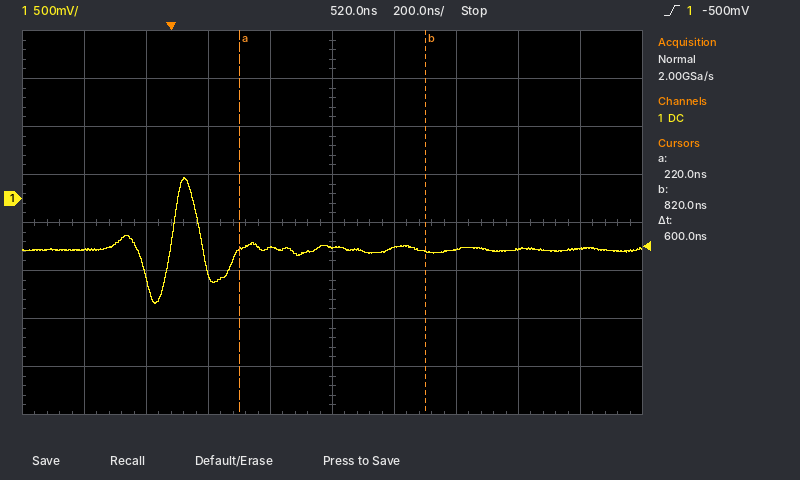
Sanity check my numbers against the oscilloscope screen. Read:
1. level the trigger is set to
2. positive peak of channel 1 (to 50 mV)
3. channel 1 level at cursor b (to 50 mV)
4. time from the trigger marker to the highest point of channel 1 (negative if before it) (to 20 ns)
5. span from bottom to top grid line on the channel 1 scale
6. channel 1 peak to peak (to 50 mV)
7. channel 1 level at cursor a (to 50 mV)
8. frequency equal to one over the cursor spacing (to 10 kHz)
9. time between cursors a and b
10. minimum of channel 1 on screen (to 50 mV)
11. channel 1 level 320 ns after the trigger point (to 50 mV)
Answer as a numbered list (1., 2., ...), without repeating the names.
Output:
1. -500 mV
2. 200 mV
3. -550 mV
4. +40 ns
5. 4 V
6. 1.30 V
7. -550 mV
8. 1.67 MHz
9. 600 ns
10. -1.10 V
11. -500 mV
